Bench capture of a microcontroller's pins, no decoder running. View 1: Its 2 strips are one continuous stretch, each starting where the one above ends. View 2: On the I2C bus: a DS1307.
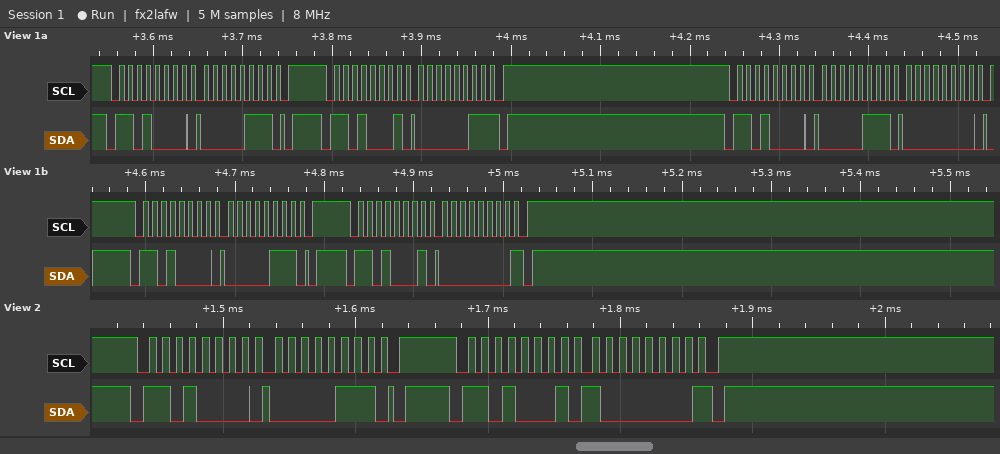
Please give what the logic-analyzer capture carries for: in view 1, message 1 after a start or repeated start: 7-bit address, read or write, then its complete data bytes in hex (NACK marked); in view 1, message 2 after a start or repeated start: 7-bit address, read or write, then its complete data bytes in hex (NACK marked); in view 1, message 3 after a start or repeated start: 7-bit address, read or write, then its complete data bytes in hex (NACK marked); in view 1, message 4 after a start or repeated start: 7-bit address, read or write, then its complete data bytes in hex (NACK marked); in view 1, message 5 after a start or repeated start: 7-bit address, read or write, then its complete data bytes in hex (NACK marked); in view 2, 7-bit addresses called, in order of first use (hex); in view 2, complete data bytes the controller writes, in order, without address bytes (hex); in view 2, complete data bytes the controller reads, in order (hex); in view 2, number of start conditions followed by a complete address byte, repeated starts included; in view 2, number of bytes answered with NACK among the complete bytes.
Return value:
0x68 write: 07
0x68 read: 03 NACK
0x68 write: 07 00
0x68 write: 07
0x68 read: 00 NACK
0x68
07
80
2
1
